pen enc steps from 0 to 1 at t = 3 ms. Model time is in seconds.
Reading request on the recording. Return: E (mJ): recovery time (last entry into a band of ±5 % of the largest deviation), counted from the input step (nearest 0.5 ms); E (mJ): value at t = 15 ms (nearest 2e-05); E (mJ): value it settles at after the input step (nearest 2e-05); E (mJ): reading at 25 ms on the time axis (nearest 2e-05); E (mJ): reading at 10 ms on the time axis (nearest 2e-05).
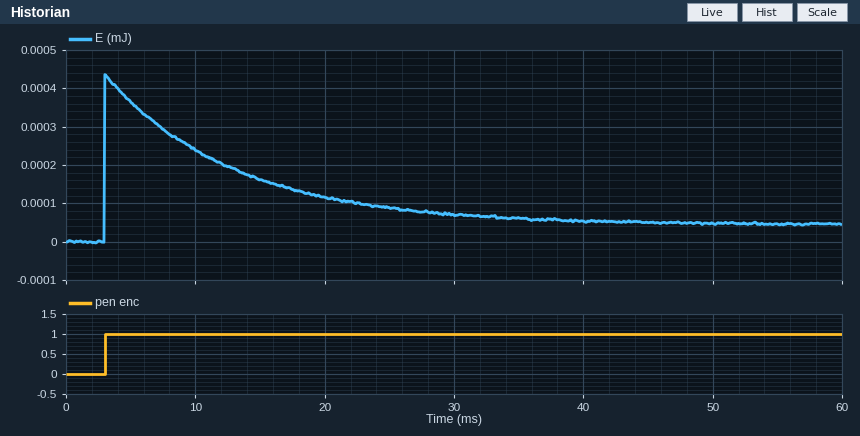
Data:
29.0 ms
0.00016
0.00004
0.00008
0.00024
